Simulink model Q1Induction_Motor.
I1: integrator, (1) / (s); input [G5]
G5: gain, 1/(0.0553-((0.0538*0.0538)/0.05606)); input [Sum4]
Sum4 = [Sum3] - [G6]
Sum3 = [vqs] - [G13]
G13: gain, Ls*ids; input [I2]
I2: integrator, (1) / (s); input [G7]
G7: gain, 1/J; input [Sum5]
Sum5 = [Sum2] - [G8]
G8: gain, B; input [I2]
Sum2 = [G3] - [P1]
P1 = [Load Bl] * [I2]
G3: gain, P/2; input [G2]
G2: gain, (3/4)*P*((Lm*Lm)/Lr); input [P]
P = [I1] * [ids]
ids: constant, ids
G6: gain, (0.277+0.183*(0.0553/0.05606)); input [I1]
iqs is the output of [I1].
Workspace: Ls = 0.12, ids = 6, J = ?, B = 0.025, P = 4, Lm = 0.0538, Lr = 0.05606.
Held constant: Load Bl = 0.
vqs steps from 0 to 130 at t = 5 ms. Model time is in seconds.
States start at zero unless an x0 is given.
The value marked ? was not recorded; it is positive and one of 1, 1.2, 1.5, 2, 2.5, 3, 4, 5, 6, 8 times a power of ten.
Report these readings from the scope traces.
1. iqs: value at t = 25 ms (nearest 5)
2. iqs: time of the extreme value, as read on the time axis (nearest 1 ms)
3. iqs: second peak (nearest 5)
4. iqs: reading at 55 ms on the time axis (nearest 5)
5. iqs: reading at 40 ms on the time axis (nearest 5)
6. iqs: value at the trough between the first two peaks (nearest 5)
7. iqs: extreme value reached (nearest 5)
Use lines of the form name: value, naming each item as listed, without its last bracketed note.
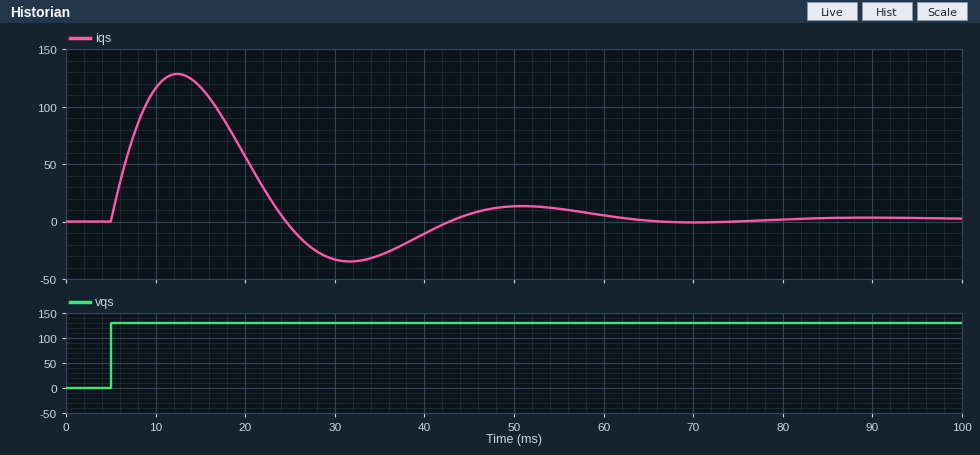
iqs: value at t = 25 ms: -5
iqs: time of the extreme value, as read on the time axis: 12 ms
iqs: second peak: 15
iqs: reading at 55 ms on the time axis: 10
iqs: reading at 40 ms on the time axis: -10
iqs: value at the trough between the first two peaks: -35
iqs: extreme value reached: 130
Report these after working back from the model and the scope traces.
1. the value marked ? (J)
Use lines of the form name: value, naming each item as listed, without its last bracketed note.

the value marked ?: 0.012
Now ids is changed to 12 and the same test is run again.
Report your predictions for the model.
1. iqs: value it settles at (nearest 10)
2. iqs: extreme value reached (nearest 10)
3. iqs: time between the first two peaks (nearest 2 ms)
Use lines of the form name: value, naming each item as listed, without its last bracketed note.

iqs: value it settles at: 0
iqs: extreme value reached: 80
iqs: time between the first two peaks: 18 ms
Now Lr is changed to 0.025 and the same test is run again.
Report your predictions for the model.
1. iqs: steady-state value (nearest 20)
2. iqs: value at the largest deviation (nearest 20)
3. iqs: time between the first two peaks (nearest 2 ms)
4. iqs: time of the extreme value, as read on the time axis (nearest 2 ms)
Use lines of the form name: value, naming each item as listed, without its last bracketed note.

iqs: steady-state value: 0
iqs: value at the largest deviation: 100
iqs: time between the first two peaks: 24 ms
iqs: time of the extreme value, as read on the time axis: 10 ms
